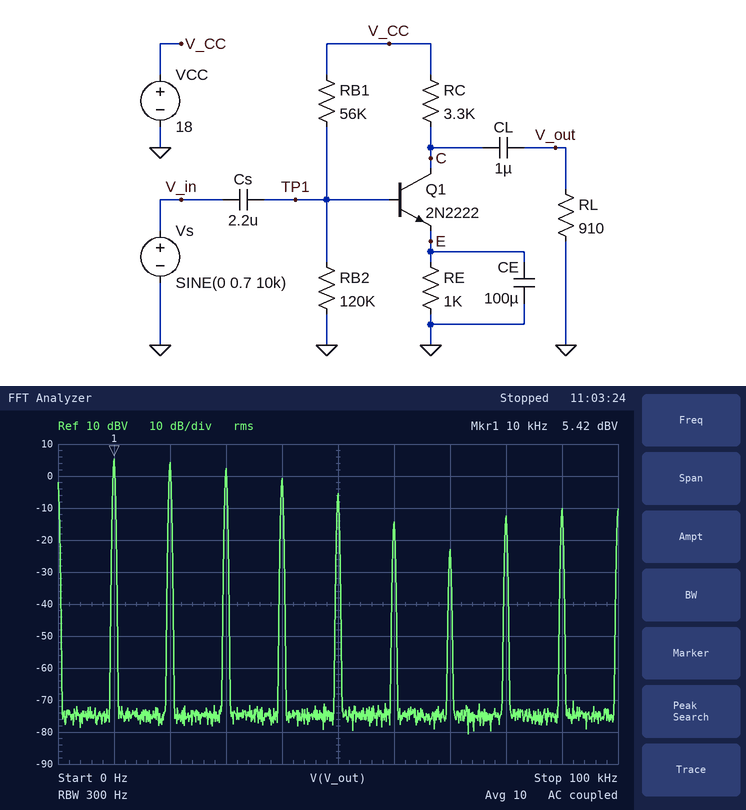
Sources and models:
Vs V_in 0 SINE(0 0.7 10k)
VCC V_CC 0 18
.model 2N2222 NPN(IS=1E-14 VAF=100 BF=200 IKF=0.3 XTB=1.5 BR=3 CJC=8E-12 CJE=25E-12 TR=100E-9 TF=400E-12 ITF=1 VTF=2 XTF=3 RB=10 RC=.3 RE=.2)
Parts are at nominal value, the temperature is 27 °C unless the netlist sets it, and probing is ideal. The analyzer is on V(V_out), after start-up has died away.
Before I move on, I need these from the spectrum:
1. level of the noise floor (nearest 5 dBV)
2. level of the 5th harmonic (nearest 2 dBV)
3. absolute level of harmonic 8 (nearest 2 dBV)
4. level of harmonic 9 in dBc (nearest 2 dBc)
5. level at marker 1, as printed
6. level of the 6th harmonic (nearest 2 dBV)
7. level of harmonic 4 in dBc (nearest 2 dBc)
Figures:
-75 dBV
-6 dBV
-12 dBV
-16 dBc
5.42 dBV
-14 dBV
-6 dBc
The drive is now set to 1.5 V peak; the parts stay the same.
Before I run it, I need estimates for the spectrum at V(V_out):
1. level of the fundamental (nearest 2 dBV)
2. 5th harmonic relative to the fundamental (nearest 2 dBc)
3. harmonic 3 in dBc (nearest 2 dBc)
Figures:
4 dBV
-6 dBc
-2 dBc
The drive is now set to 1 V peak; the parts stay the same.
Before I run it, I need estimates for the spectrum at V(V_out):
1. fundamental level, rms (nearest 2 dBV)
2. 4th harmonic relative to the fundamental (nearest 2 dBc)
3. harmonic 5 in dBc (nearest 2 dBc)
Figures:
4 dBV
-4 dBc
-8 dBc
